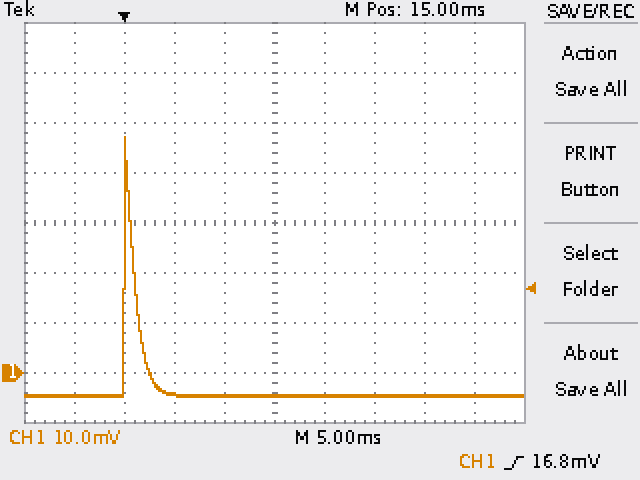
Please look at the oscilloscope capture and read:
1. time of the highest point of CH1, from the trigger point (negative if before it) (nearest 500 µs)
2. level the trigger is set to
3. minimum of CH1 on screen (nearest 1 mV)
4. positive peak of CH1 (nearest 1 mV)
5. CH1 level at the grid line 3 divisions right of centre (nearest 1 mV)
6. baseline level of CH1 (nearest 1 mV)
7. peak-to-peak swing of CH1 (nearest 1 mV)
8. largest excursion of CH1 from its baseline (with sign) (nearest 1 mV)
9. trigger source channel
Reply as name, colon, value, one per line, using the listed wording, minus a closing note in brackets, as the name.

time of the highest point of CH1, from the trigger point (negative if before it): 0.0 ms
level the trigger is set to: 16.8 mV
minimum of CH1 on screen: -5 mV
positive peak of CH1: 47 mV
CH1 level at the grid line 3 divisions right of centre: -5 mV
baseline level of CH1: -5 mV
peak-to-peak swing of CH1: 52 mV
largest excursion of CH1 from its baseline (with sign): +52 mV
trigger source channel: CH1
